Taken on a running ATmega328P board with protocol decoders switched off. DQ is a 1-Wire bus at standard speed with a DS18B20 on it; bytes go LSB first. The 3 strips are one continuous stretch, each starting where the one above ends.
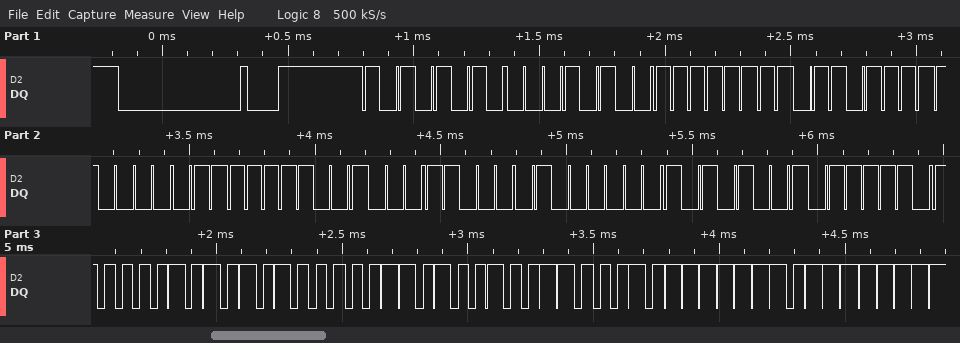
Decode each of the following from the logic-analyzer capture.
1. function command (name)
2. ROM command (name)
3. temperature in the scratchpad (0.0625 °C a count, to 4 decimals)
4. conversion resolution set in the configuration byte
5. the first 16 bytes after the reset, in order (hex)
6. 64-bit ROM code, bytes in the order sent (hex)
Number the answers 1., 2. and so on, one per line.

1. Read Scratchpad
2. Match ROM
3. 85.0000 °C
4. 12 bits
5. 55 28 FF F6 C1 9F 18 02 95 BE 50 05 4B 46 7F FF
6. 28 FF F6 C1 9F 18 02 95
